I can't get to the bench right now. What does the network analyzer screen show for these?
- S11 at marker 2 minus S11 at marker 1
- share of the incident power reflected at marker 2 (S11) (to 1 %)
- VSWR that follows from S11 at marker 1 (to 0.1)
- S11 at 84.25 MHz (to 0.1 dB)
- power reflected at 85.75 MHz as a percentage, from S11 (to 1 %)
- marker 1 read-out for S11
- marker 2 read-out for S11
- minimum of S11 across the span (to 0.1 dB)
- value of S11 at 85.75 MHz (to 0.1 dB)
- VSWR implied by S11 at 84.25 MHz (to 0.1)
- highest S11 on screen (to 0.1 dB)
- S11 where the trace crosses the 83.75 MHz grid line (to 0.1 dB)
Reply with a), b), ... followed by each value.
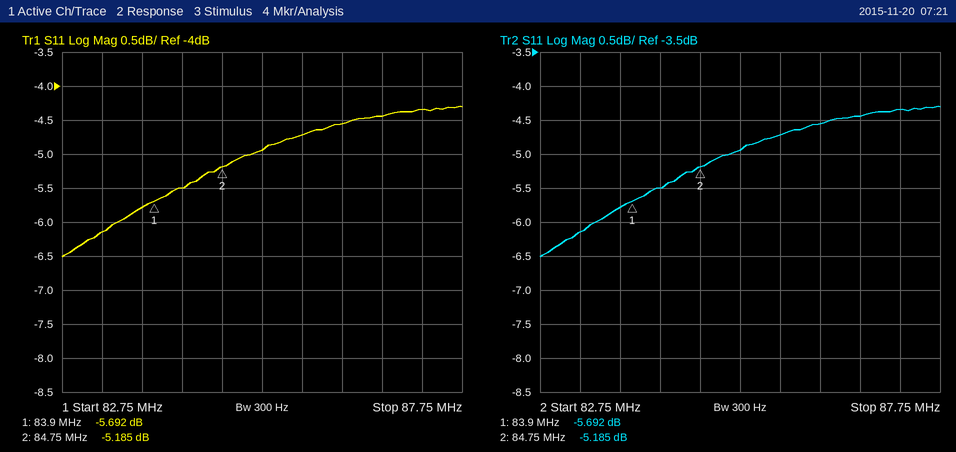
a) 0.507 dB
b) 30 %
c) 3.2
d) -5.5 dB
e) 34 %
f) -5.692 dB
g) -5.185 dB
h) -6.5 dB
i) -4.7 dB
j) 3.3
k) -4.3 dB
l) -5.8 dB
